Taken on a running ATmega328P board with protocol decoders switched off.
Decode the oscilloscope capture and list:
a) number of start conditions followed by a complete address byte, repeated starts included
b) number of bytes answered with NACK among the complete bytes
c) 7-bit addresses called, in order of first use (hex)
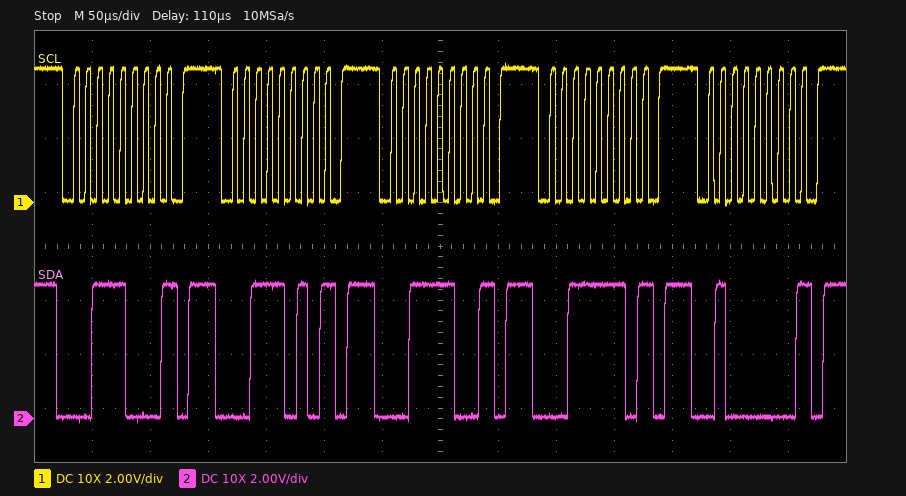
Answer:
5
5
0x1C 0x1D 0x1E 0x1F 0x20
